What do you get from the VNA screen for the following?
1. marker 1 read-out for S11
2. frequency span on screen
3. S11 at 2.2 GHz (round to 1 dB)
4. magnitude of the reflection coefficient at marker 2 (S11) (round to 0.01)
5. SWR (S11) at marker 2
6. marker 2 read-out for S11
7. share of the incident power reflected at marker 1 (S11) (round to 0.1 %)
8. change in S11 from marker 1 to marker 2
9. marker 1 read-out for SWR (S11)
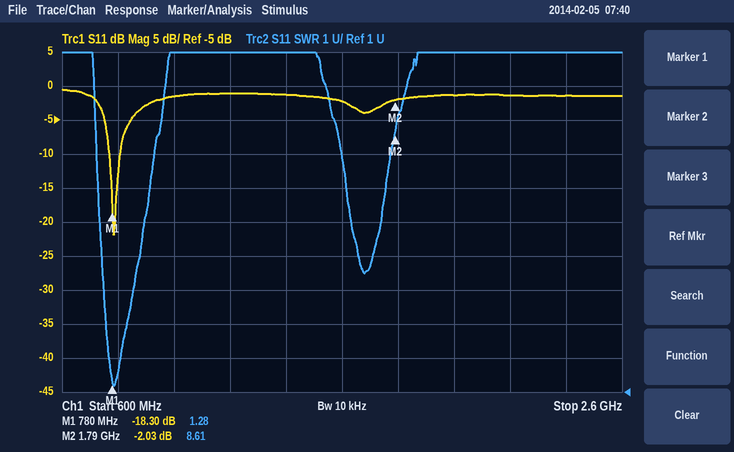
-18.30 dB
2 GHz
-1 dB
0.79
8.61
-2.03 dB
1.5 %
16.27 dB
1.28
